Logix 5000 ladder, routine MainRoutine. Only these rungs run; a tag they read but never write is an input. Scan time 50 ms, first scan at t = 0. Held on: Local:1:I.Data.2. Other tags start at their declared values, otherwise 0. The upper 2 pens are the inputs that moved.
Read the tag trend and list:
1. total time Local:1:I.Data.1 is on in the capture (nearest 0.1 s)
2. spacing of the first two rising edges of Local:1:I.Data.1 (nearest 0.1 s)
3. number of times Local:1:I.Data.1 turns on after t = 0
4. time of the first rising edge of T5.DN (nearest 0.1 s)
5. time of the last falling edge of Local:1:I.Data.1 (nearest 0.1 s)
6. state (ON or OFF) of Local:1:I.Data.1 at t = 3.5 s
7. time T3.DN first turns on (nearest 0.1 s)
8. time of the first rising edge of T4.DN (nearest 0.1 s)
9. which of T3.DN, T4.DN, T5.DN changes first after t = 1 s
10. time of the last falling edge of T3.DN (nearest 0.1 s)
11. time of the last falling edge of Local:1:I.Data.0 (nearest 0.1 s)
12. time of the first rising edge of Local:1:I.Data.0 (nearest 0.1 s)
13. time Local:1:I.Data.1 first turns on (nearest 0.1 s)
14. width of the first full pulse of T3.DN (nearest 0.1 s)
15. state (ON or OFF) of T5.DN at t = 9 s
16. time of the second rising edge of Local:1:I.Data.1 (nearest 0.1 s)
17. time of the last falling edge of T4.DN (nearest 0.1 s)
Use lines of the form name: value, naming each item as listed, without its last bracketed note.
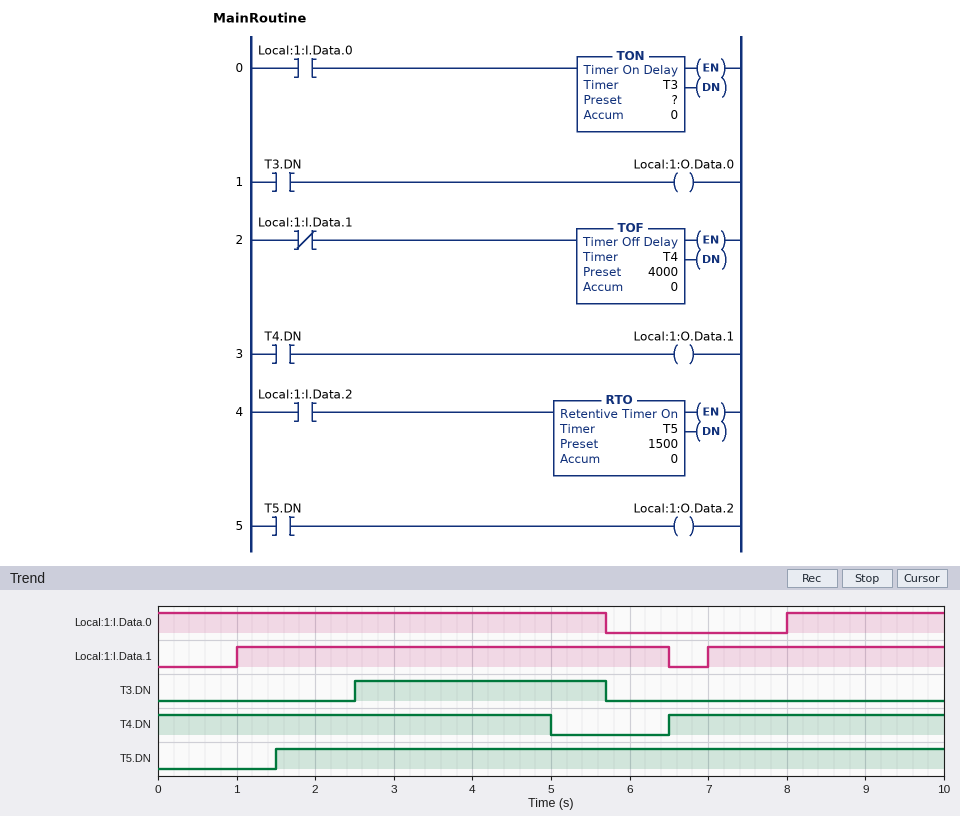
total time Local:1:I.Data.1 is on in the capture: 8.5 s
spacing of the first two rising edges of Local:1:I.Data.1: 6.0 s
number of times Local:1:I.Data.1 turns on after t = 0: 2
time of the first rising edge of T5.DN: 1.5 s
time of the last falling edge of Local:1:I.Data.1: 6.5 s
state (ON or OFF) of Local:1:I.Data.1 at t = 3.5 s: ON
time T3.DN first turns on: 2.5 s
time of the first rising edge of T4.DN: 6.5 s
which of T3.DN, T4.DN, T5.DN changes first after t = 1 s: T5.DN
time of the last falling edge of T3.DN: 5.7 s
time of the last falling edge of Local:1:I.Data.0: 5.7 s
time of the first rising edge of Local:1:I.Data.0: 8.0 s
time Local:1:I.Data.1 first turns on: 1.0 s
width of the first full pulse of T3.DN: 3.2 s
state (ON or OFF) of T5.DN at t = 9 s: ON
time of the second rising edge of Local:1:I.Data.1: 7.0 s
time of the last falling edge of T4.DN: 5.0 s
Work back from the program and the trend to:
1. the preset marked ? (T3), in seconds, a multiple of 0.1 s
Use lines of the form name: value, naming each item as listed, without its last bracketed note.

the preset marked ? (T3), in seconds, a multiple of 0.1 s: 2.5 s
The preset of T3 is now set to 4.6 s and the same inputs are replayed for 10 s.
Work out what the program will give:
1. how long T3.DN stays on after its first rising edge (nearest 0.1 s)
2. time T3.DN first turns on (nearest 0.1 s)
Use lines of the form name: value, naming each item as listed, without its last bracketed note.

how long T3.DN stays on after its first rising edge: 1.1 s
time T3.DN first turns on: 4.6 s
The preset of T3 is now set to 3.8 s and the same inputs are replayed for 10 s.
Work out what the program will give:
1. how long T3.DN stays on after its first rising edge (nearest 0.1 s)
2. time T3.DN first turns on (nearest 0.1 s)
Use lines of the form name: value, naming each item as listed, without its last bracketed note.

how long T3.DN stays on after its first rising edge: 1.9 s
time T3.DN first turns on: 3.8 s
